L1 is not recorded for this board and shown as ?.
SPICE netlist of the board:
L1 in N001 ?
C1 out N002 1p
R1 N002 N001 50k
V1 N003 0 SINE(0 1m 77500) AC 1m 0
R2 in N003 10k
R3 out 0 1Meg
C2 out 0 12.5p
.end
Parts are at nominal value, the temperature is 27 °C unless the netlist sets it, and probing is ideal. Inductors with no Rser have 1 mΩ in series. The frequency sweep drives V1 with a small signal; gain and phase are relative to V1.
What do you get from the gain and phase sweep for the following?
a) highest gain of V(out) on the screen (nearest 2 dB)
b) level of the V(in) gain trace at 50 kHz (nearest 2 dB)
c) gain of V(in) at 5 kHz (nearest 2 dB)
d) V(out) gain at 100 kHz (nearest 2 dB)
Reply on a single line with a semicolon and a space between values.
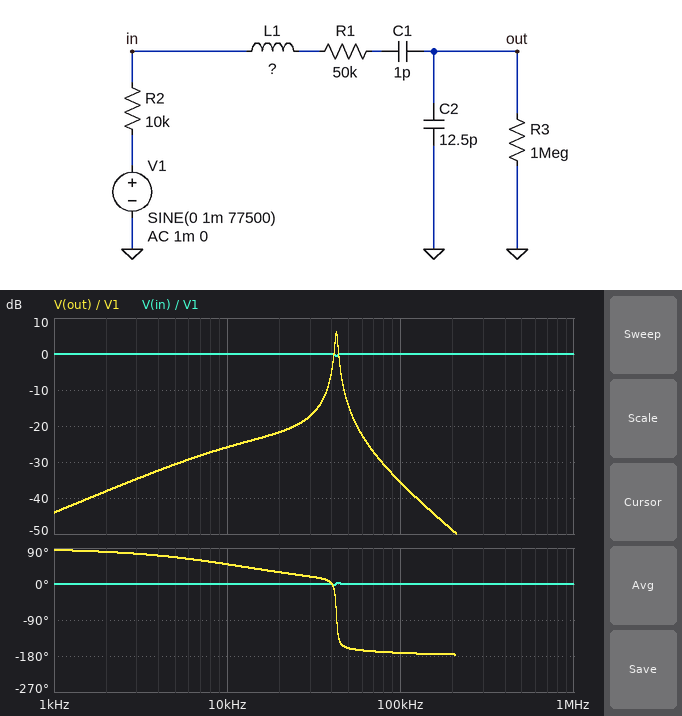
6 dB; 0 dB; 0 dB; -36 dB
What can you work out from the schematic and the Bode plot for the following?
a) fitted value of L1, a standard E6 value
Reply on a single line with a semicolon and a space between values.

15 H
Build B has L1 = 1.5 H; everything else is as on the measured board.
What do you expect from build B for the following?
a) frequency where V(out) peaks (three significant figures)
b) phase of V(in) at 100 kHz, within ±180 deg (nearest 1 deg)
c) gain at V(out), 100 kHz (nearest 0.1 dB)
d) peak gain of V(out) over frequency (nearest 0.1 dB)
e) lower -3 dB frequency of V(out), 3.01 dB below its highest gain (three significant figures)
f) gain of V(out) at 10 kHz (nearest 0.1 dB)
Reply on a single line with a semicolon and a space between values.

135 kHz; -1 deg; -15.8 dB; 2.7 dB; 131 kHz; -26.3 dB
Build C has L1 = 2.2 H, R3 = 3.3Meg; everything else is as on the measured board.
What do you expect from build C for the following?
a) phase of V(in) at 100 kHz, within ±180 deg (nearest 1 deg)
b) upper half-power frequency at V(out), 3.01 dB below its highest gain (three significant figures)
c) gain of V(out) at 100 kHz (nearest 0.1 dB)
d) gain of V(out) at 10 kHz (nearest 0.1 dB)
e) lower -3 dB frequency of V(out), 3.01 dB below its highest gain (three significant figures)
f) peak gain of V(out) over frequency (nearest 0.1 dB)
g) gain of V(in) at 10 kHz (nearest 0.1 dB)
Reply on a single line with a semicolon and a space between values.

-2 deg; 114 kHz; -8.6 dB; -23.1 dB; 109 kHz; 5.0 dB; 0 dB
